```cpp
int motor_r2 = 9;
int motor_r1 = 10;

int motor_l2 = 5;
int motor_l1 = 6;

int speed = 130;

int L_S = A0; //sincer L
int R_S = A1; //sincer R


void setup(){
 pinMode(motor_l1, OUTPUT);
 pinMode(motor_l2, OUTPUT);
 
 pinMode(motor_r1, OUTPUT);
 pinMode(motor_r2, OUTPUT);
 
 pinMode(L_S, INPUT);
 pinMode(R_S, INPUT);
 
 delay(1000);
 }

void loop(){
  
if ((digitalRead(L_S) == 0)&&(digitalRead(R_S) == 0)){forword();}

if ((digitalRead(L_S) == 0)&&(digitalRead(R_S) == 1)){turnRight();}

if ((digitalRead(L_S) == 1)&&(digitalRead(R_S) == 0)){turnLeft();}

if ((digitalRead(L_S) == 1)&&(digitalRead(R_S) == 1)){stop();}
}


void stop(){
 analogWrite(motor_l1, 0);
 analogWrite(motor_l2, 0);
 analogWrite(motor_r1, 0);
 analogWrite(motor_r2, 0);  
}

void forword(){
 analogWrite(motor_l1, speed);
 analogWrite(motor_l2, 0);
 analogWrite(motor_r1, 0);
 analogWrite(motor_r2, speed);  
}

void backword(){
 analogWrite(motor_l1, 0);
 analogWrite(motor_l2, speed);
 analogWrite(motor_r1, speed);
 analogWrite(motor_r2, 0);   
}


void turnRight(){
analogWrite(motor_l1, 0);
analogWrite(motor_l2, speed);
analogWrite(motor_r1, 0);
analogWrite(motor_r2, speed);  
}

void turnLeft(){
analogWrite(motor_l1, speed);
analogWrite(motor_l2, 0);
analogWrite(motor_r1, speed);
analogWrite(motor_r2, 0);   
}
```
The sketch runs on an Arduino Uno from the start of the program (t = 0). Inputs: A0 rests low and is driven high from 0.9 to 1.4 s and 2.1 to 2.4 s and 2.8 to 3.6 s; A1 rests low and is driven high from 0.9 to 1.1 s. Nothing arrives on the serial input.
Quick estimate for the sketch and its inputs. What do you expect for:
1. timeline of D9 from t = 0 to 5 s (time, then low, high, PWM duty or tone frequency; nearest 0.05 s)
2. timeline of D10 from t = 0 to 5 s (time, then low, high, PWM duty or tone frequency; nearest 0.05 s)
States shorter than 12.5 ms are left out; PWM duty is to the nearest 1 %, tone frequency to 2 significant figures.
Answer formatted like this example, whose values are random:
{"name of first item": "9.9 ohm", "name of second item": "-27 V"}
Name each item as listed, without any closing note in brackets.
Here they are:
{"timeline of D9 from t = 0 to 5 s": "0 s low; 1.4 s PWM 51 %; 2.1 s low; 2.4 s PWM 51 %; 2.8 s low; 3.6 s PWM 51 %", "timeline of D10 from t = 0 to 5 s": "0 s low; 1.1 s PWM 51 %; 1.4 s low; 2.1 s PWM 51 %; 2.4 s low; 2.8 s PWM 51 %; 3.6 s low"}
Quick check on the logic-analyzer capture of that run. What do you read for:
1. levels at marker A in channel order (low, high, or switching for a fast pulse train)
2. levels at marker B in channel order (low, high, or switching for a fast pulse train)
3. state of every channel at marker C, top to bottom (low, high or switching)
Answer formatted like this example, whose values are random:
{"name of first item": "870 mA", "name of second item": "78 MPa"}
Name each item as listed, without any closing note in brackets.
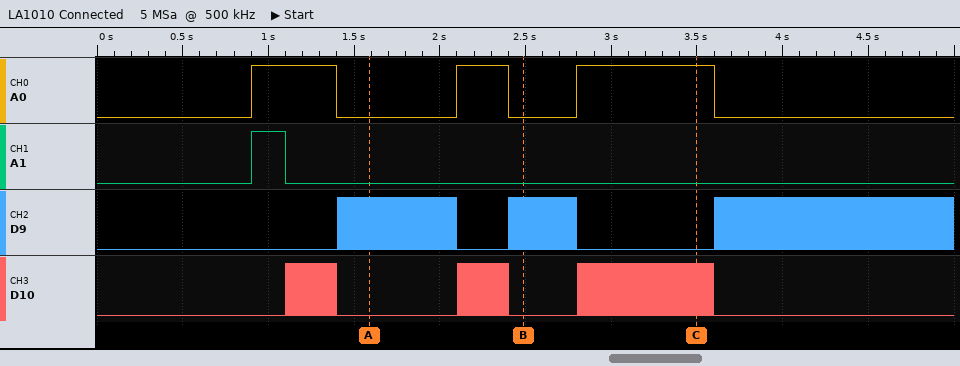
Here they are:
{"levels at marker A in channel order": "A0 low, A1 low, D9 switching, D10 low", "levels at marker B in channel order": "A0 low, A1 low, D9 switching, D10 low", "state of every channel at marker C, top to bottom": "A0 high, A1 low, D9 low, D10 switching"}
